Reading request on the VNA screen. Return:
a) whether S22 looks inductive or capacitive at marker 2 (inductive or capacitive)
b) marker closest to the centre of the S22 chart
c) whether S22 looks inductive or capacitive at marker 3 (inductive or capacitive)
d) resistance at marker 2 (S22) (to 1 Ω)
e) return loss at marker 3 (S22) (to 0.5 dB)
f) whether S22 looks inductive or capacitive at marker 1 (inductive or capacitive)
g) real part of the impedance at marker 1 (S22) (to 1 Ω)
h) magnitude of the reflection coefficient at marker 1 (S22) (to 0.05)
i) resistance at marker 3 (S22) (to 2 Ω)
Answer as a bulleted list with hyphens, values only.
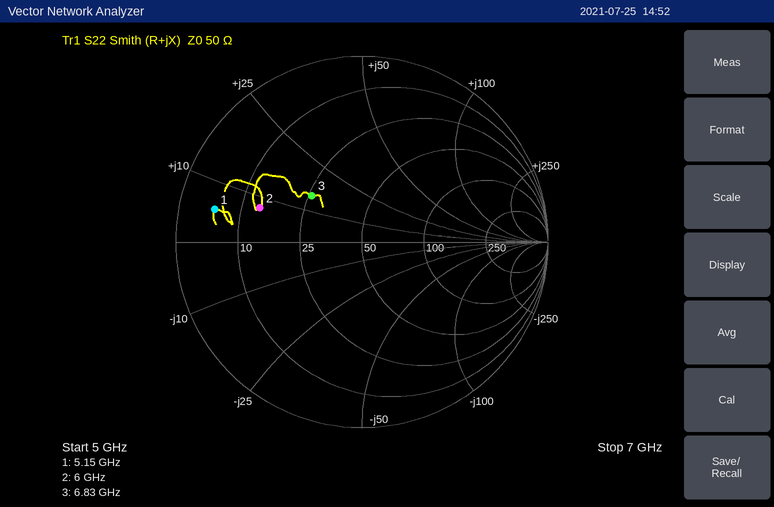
- inductive
- marker 3
- inductive
- 14 Ω
- 8.5 dB
- inductive
- 5 Ω
- 0.80
- 26 Ω
